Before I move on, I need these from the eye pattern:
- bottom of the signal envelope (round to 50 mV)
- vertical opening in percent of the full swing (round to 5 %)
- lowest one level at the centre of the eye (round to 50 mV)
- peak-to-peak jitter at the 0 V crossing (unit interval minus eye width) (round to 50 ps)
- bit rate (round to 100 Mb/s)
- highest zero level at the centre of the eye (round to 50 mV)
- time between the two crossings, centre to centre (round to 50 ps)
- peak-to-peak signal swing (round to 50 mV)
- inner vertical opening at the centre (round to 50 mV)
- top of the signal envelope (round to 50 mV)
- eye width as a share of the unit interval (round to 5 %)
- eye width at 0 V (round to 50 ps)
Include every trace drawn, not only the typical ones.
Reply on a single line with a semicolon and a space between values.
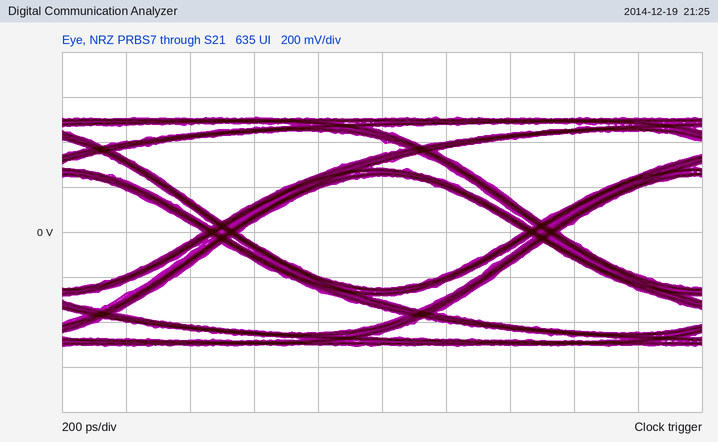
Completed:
-500 mV; 50 %; 250 mV; 100 ps; 1.0 Gb/s; -250 mV; 1.00 ns; 1.00 V; 500 mV; 500 mV; 90 %; 900 ps
